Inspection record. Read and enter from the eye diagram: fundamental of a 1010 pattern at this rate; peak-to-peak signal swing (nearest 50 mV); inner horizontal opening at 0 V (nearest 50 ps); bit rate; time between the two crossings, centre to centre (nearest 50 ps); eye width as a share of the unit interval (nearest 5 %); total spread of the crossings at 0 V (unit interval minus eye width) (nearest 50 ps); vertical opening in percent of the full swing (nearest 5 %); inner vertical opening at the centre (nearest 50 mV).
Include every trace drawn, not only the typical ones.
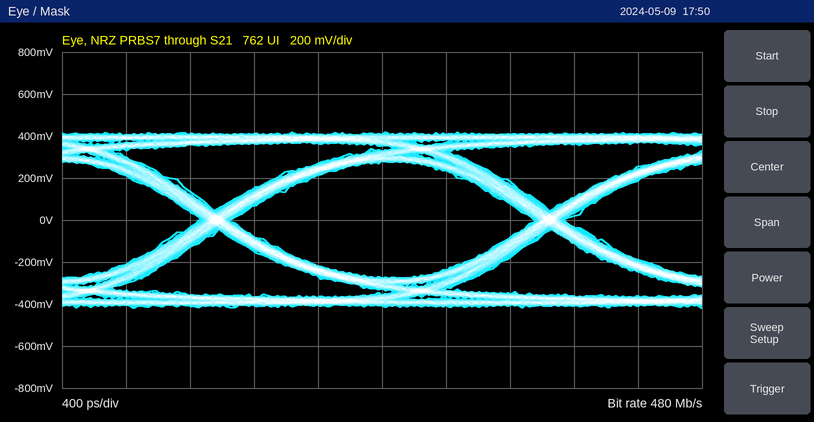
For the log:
240 MHz
850 mV
1.90 ns
480 Mb/s
2.10 ns
90 %
200 ps
65 %
550 mV
